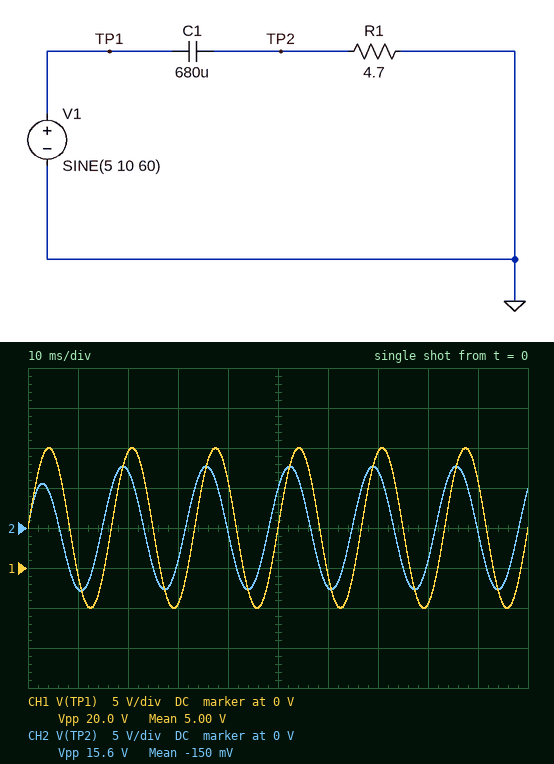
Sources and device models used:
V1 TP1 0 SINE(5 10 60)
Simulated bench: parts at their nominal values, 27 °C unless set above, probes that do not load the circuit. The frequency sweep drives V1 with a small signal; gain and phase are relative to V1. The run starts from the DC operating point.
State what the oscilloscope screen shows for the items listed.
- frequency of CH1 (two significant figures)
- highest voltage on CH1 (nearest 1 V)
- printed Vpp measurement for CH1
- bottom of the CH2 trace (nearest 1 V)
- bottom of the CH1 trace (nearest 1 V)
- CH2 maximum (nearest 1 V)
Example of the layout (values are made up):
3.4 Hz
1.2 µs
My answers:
60 Hz
15 V
20.0 V
-8 V
-5 V
8 V
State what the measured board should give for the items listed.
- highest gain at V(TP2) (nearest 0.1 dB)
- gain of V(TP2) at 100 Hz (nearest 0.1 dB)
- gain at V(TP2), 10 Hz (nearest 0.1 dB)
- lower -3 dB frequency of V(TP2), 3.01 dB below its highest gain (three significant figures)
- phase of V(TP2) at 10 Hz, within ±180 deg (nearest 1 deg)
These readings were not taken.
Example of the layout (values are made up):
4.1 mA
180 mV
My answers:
0 dB
-1.0 dB
-14.1 dB
49.8 Hz
79 deg
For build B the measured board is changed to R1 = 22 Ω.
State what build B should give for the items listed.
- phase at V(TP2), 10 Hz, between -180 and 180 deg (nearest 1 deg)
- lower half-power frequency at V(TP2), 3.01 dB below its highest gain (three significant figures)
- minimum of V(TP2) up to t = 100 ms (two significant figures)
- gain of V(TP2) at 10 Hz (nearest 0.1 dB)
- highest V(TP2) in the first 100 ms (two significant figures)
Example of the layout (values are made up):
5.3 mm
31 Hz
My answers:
47 deg
10.6 Hz
-11 V
-3.3 dB
9.8 V
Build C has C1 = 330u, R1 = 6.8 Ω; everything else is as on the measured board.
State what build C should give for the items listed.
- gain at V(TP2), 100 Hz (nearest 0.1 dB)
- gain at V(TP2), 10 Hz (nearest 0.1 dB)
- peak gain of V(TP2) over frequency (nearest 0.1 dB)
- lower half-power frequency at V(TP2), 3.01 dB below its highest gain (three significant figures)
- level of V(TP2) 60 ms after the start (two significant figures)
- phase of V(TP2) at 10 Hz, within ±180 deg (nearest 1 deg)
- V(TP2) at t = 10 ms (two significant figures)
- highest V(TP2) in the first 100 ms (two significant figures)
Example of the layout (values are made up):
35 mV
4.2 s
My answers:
-1.8 dB
-17.1 dB
0 dB
70.9 Hz
-6.4 V
82 deg
-6.5 V
6.5 V
